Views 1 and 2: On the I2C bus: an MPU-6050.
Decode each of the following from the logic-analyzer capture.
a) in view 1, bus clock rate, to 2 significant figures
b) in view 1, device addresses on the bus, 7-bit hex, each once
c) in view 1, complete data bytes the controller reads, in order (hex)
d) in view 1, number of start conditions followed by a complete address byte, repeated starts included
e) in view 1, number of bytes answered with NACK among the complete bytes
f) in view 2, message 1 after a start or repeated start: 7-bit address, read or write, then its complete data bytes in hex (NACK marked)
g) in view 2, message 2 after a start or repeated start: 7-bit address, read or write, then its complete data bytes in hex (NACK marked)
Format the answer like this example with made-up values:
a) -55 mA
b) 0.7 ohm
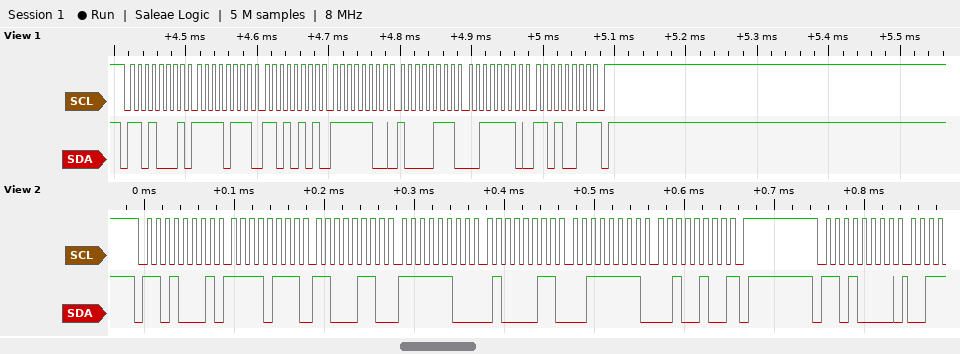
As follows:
a) 100 kHz
b) 0x68
c) F7 D5 FC 87 3E D3
d) 1
e) 1
f) 0x68 read: F7 C6 FC 43 3F 24 NACK
g) 0x68 write
